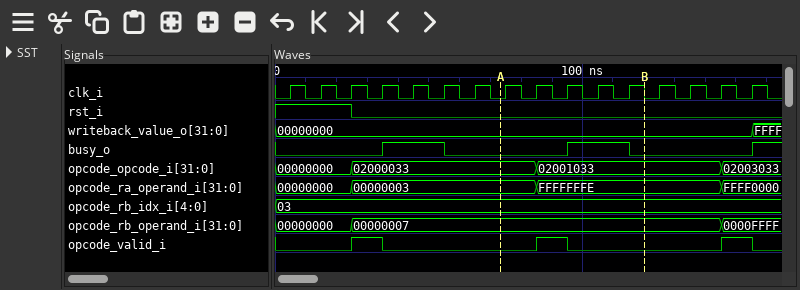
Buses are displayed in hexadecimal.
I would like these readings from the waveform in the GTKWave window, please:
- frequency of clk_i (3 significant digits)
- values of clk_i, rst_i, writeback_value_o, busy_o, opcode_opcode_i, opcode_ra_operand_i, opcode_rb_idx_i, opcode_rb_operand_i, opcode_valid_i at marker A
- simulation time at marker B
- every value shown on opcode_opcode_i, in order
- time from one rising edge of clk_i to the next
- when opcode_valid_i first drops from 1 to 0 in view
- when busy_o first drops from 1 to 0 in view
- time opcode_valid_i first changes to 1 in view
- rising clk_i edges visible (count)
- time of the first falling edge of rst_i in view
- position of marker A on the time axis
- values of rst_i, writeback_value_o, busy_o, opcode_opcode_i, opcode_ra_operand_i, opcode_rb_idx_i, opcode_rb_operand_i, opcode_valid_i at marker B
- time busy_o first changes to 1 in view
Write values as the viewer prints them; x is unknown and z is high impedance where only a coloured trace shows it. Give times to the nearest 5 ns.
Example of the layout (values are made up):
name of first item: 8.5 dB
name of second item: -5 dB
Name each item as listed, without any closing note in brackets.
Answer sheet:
frequency of clk_i: 100 MHz
values of clk_i, rst_i, writeback_value_o, busy_o, opcode_opcode_i, opcode_ra_operand_i, opcode_rb_idx_i, opcode_rb_operand_i, opcode_valid_i at marker A: clk_i=0, rst_i=0, writeback_value_o=00000000, busy_o=0, opcode_opcode_i=02000033, opcode_ra_operand_i=00000003, opcode_rb_idx_i=03, opcode_rb_operand_i=00000007, opcode_valid_i=0
simulation time at marker B: 120 ns
every value shown on opcode_opcode_i, in order: 00000000, 02000033, 02001033, 02003033
time from one rising edge of clk_i to the next: 10 ns
when opcode_valid_i first drops from 1 to 0 in view: 35 ns
when busy_o first drops from 1 to 0 in view: 55 ns
time opcode_valid_i first changes to 1 in view: 25 ns
rising clk_i edges visible: 16
time of the first falling edge of rst_i in view: 25 ns
position of marker A on the time axis: 75 ns
values of rst_i, writeback_value_o, busy_o, opcode_opcode_i, opcode_ra_operand_i, opcode_rb_idx_i, opcode_rb_operand_i, opcode_valid_i at marker B: rst_i=0, writeback_value_o=00000000, busy_o=0, opcode_opcode_i=02001033, opcode_ra_operand_i=FFFFFFFE, opcode_rb_idx_i=03, opcode_rb_operand_i=00000007, opcode_valid_i=0
time busy_o first changes to 1 in view: 35 ns
